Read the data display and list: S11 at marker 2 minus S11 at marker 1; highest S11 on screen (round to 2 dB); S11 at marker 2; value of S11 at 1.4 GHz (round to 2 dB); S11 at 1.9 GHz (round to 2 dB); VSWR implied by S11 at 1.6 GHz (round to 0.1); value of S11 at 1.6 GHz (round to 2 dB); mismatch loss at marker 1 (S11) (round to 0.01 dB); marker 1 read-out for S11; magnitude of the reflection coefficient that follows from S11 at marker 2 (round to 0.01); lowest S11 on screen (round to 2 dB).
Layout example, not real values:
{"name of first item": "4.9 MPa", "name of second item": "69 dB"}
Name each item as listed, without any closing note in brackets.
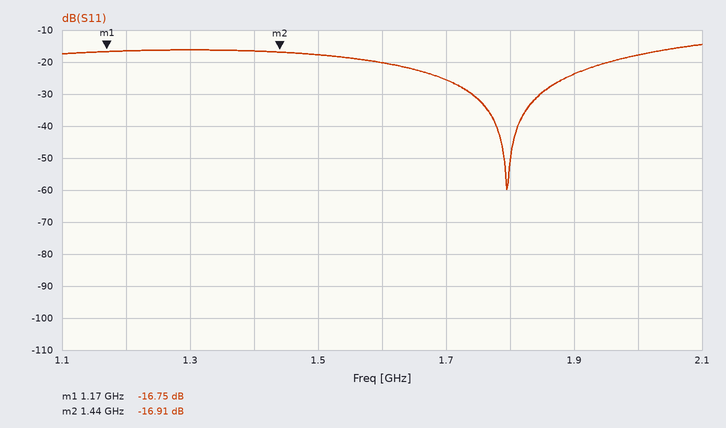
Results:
{"S11 at marker 2 minus S11 at marker 1": "-0.16 dB", "highest S11 on screen": "-14 dB", "S11 at marker 2": "-16.91 dB", "value of S11 at 1.4 GHz": "-16 dB", "S11 at 1.9 GHz": "-24 dB", "VSWR implied by S11 at 1.6 GHz": "1.2", "value of S11 at 1.6 GHz": "-20 dB", "mismatch loss at marker 1 (S11)": "0.09 dB", "marker 1 read-out for S11": "-16.75 dB", "magnitude of the reflection coefficient that follows from S11 at marker 2": "0.14", "lowest S11 on screen": "-60 dB"}
